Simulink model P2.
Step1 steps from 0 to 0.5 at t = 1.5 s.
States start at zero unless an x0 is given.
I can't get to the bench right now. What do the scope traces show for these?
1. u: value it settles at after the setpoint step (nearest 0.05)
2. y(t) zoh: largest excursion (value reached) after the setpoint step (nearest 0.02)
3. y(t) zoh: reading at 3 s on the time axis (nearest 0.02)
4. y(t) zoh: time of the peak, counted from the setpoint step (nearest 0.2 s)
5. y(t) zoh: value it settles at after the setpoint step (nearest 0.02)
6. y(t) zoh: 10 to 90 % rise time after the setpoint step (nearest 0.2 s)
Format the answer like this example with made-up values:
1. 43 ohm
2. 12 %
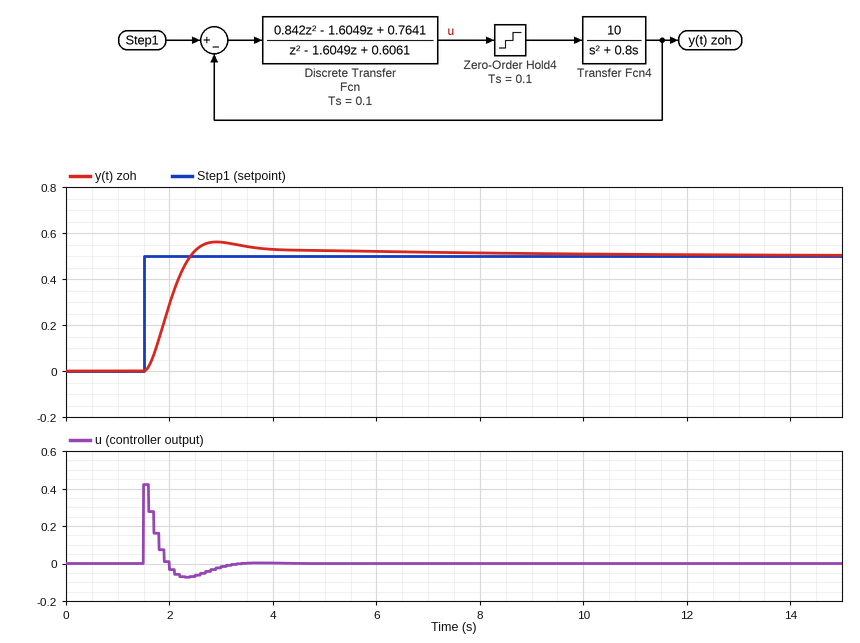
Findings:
1. 0.00
2. 0.56
3. 0.56
4. 1.4 s
5. 0.50
6. 0.6 s
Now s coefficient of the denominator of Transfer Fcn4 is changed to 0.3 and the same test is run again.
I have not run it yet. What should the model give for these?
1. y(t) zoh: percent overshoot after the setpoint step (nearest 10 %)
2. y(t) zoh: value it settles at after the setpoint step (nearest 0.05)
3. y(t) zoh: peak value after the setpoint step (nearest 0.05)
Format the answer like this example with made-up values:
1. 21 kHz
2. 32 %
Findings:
1. 30 %
2. 0.50
3. 0.65
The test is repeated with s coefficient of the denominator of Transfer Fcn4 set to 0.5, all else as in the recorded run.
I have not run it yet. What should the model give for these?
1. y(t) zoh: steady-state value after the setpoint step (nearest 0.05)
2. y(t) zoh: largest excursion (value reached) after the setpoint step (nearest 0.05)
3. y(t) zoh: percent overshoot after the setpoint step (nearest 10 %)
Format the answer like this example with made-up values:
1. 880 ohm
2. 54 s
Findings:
1. 0.50
2. 0.60
3. 20 %
